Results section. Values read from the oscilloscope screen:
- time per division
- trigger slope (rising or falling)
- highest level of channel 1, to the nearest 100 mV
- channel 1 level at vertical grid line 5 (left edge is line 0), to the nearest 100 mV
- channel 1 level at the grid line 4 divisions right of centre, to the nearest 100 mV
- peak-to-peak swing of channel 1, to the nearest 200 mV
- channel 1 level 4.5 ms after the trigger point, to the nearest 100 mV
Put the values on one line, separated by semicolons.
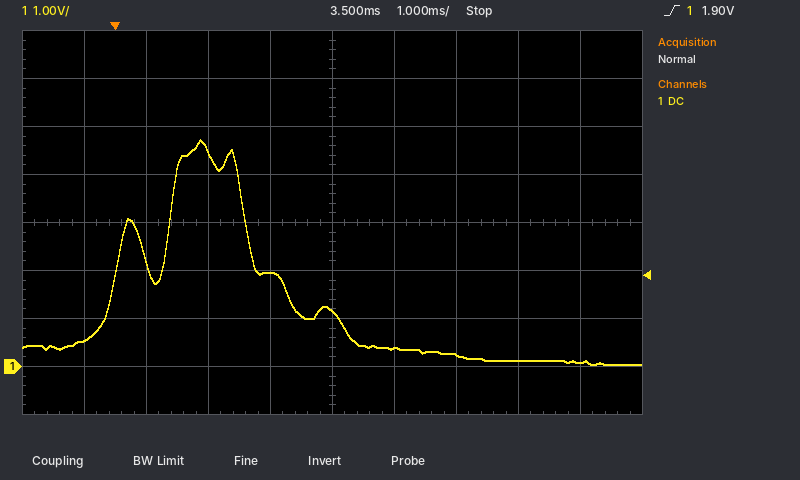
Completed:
1 ms; rising; 4.7 V; 1.2 V; 100 mV; 4.6 V; 400 mV
